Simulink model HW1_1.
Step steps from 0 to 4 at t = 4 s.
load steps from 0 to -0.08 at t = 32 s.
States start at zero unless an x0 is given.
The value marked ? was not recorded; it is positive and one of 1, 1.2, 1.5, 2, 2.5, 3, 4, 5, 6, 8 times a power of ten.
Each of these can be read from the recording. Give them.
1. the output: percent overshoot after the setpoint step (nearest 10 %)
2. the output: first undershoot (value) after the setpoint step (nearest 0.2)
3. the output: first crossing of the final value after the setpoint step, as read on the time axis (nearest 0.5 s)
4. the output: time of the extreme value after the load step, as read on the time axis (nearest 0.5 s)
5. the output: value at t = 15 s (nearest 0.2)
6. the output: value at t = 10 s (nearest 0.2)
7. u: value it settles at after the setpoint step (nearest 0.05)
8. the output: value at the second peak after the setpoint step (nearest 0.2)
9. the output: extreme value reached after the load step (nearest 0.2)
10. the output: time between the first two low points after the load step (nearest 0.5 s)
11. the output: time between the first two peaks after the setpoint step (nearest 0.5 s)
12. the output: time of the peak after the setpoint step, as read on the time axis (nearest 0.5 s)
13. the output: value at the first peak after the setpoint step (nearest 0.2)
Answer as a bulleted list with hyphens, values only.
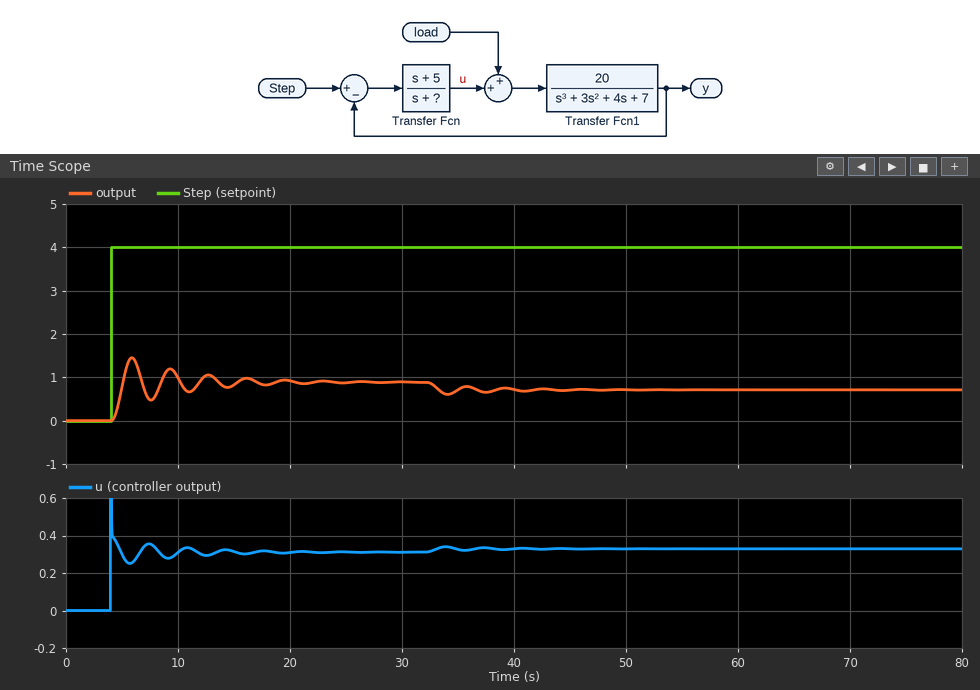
- 60 %
- 0.4
- 5.0 s
- 34.0 s
- 0.8
- 1.0
- 0.30
- 1.2
- 0.6
- 3.5 s
- 3.5 s
- 6.0 s
- 1.4
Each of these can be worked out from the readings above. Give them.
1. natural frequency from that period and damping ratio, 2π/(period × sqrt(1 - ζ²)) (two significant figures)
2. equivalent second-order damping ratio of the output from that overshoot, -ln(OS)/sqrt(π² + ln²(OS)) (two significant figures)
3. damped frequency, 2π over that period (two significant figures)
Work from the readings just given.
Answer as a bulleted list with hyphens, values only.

- 1.8 rad/s
- 0.16
- 1.8 rad/s
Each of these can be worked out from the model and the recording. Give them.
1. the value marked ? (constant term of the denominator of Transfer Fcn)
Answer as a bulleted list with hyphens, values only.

- 50
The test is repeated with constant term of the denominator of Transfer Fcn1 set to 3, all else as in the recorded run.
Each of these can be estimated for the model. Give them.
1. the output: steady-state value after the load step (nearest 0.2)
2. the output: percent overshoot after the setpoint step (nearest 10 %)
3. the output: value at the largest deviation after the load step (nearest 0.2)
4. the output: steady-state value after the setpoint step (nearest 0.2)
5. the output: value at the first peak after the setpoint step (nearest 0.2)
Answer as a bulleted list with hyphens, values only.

- 1.2
- 30 %
- 1.2
- 1.6
- 2.0
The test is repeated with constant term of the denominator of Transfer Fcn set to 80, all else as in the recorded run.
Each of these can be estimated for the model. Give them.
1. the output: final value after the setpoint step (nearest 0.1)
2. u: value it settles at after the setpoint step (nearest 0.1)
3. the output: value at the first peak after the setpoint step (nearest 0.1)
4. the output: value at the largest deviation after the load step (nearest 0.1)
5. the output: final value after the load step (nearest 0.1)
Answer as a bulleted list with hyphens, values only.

- 0.6
- 0.2
- 1.0
- 0.3
- 0.4
